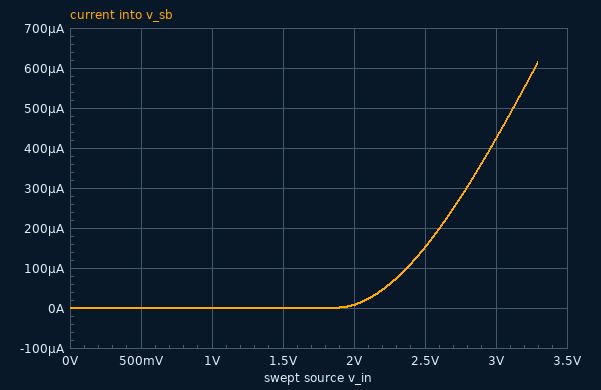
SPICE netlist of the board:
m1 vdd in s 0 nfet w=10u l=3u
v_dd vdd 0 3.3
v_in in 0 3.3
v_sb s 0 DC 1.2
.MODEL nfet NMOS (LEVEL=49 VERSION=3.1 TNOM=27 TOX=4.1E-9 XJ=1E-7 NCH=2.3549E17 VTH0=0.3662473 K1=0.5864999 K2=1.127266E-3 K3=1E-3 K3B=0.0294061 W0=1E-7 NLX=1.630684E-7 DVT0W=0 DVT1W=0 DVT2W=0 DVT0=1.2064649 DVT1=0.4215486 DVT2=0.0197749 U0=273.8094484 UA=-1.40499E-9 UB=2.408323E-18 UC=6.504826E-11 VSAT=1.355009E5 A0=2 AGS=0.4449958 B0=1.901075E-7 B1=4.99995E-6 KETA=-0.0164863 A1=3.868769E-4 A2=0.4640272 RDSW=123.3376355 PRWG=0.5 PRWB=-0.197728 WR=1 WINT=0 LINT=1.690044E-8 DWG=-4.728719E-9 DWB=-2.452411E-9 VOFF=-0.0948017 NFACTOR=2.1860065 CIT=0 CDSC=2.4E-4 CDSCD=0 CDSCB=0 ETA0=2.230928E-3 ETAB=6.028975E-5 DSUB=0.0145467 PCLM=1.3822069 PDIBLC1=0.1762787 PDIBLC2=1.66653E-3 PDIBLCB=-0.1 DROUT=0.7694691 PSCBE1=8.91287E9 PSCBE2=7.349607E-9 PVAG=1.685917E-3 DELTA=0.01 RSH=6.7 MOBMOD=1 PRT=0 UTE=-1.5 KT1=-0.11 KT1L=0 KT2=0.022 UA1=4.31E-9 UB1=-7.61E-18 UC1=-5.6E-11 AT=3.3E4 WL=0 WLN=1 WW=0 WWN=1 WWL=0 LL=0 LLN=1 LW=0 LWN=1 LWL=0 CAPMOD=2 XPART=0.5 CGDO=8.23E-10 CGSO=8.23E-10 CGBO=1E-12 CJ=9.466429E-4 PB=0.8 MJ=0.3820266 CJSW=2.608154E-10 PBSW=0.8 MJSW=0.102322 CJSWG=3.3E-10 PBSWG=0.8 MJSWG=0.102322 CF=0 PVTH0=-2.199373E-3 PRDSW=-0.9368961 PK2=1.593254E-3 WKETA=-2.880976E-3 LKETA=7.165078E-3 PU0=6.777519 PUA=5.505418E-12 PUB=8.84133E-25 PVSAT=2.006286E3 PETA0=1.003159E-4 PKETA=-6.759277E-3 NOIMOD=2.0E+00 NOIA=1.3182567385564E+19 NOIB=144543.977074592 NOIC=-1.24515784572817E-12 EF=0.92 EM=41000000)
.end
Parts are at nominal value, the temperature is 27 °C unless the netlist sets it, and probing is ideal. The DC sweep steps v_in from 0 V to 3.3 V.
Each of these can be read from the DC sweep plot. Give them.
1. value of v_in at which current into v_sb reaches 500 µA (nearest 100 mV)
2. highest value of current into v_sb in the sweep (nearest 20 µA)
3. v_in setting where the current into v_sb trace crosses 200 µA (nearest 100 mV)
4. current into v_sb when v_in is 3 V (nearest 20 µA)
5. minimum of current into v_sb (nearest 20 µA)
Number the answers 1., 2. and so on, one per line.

1. 3.1 V
2. 620 µA
3. 2.6 V
4. 420 µA
5. 0 A
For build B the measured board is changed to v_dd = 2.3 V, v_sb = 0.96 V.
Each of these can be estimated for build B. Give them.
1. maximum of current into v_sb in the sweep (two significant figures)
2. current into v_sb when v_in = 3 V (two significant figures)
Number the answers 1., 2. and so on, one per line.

1. 800 µA
2. 610 µA
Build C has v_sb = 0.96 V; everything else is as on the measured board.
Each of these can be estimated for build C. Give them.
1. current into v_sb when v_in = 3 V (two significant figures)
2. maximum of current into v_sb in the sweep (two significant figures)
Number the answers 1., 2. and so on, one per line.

1. 620 µA
2. 830 µA
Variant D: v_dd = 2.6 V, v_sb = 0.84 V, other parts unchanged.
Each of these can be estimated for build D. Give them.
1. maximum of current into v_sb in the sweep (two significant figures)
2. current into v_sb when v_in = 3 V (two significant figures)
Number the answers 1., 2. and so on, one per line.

1. 940 µA
2. 730 µA
